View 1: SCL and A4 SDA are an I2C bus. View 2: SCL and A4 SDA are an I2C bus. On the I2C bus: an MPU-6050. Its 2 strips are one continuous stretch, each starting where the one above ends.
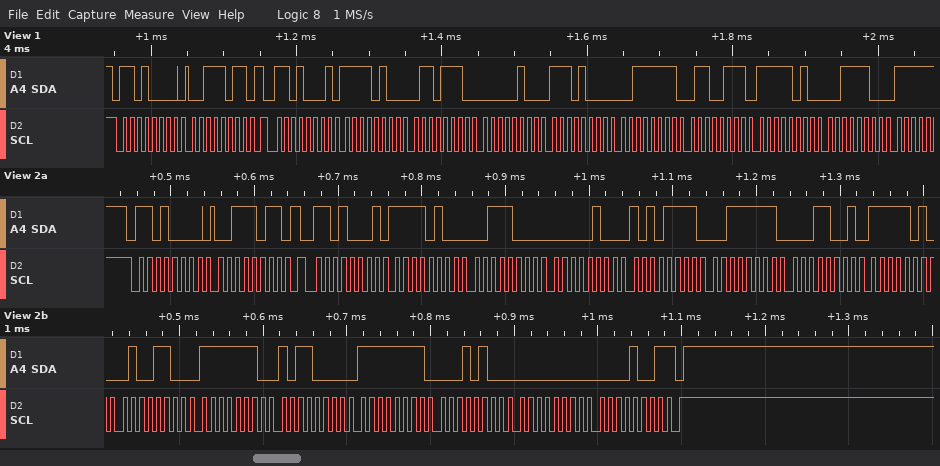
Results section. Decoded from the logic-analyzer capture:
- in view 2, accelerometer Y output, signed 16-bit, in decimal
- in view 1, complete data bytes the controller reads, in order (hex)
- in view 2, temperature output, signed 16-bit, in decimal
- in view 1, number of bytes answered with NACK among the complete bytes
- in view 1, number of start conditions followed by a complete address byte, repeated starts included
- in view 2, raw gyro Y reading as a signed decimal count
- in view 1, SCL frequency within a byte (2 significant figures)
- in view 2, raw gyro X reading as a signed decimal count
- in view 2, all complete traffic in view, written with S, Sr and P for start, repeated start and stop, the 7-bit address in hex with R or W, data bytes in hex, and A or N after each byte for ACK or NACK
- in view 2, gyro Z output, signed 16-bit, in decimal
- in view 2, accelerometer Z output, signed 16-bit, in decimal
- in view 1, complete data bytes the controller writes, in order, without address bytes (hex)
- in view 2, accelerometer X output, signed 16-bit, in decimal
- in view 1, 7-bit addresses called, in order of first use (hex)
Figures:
1199
F4 6E 04 E8 3F 67 FA 3C
-1460
0
2
-236
100 kHz
-336
S 68W A 3B A Sr 68R A F4 A 38 A 04 A AF A 3F A 19 A FA A 4C A FE A B0 A FF A 14 A 00 A 09 N P
9
16153
3B
-3016
0x68
